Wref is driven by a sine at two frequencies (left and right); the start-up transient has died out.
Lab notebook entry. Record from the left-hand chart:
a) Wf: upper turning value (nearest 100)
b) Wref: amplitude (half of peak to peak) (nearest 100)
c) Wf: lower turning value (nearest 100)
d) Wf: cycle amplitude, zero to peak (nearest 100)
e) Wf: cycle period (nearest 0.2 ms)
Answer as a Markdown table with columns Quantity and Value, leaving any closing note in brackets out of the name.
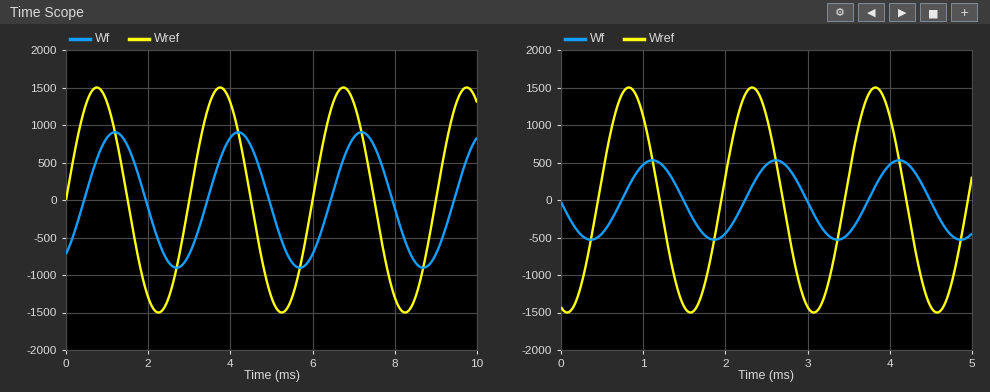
| Quantity | Value |
|---|---|
| Wf: upper turning value | 900 |
| Wref: amplitude (half of peak to peak) | 1500 |
| Wf: lower turning value | -900 |
| Wf: cycle amplitude, zero to peak | 900 |
| Wf: cycle period | 3.0 ms |
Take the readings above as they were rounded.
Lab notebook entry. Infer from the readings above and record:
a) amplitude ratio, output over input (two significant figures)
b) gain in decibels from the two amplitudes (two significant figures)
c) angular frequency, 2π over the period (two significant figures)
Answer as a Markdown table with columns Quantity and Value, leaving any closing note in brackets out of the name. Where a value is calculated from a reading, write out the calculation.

| Quantity | Value |
|---|---|
| amplitude ratio, output over input | 900 / 1500 = 0.60 |
| gain in decibels from the two amplitudes | 20 log10(900 / 1500) = -4.4 dB |
| angular frequency, 2π over the period | 2π / 3 = 2.1 rad/ms |
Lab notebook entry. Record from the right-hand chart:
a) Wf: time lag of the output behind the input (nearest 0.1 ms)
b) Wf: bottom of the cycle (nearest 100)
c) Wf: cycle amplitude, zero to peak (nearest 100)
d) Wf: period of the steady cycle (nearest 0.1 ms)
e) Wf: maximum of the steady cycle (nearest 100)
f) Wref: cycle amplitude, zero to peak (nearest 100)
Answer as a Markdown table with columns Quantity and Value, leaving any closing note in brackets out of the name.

| Quantity | Value |
|---|---|
| Wf: time lag of the output behind the input | 0.3 ms |
| Wf: bottom of the cycle | -500 |
| Wf: cycle amplitude, zero to peak | 500 |
| Wf: period of the steady cycle | 1.5 ms |
| Wf: maximum of the steady cycle | 500 |
| Wref: cycle amplitude, zero to peak | 1500 |
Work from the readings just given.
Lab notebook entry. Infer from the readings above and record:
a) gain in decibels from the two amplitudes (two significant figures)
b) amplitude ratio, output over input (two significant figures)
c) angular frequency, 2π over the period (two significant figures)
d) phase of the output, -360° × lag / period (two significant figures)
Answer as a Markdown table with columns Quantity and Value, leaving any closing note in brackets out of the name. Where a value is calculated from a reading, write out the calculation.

| Quantity | Value |
|---|---|
| gain in decibels from the two amplitudes | 20 log10(500 / 1500) = -9.5 dB |
| amplitude ratio, output over input | 500 / 1500 = 0.33 |
| angular frequency, 2π over the period | 2π / 1.5 = 4.2 rad/ms |
| phase of the output, -360° × lag / period | -360 × 0.3 / 1.5 = -72° |
